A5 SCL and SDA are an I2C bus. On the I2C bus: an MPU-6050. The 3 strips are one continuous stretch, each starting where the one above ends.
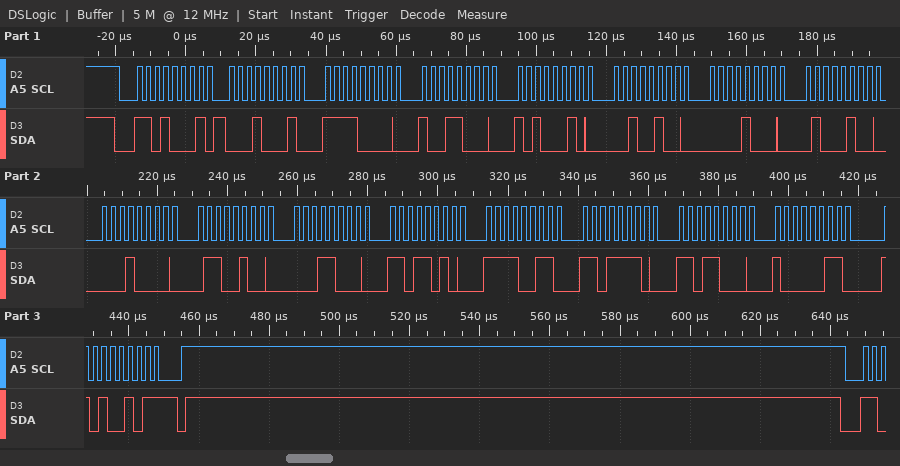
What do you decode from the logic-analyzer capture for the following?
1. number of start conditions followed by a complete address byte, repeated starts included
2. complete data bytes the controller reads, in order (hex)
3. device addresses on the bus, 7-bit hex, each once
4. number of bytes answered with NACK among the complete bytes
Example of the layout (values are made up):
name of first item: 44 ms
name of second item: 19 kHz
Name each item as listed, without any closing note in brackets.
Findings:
number of start conditions followed by a complete address byte, repeated starts included: 1
complete data bytes the controller reads, in order: 11 F0 98 A2 24 08 44 10 64 18 DA F3 DE D8 83 A5
device addresses on the bus, 7-bit hex, each once: 0x68
number of bytes answered with NACK among the complete bytes: 1
